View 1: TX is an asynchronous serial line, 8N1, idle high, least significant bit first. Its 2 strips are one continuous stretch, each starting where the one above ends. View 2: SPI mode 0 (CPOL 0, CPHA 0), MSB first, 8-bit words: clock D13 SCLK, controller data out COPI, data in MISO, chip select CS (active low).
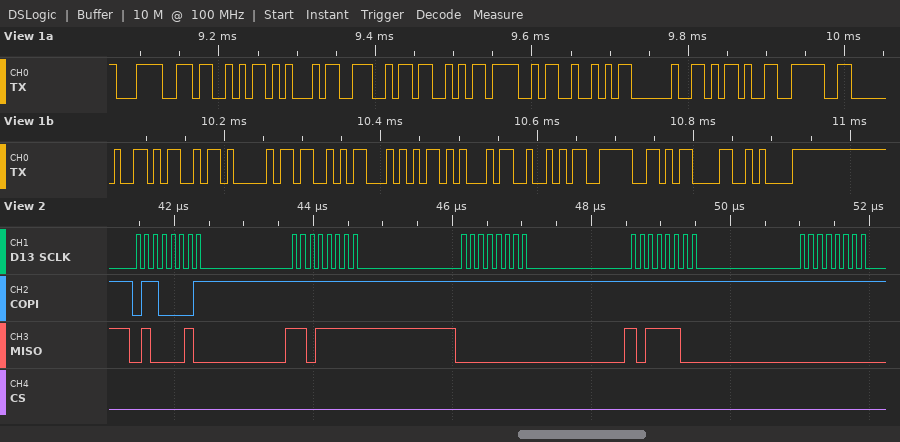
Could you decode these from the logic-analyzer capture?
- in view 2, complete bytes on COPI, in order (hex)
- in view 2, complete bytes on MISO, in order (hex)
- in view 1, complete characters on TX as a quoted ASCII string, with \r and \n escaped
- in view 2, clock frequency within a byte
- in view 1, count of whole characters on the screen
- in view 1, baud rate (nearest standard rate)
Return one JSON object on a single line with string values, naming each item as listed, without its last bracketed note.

{"in view 2, complete bytes on COPI, in order": "61 FF FF FF FF", "in view 2, complete bytes on MISO, in order": "42 DF 00 BC 00", "in view 1, complete characters on TX as a quoted ASCII string, with \\r and \\n escaped": "\"<SENSOR -> MASTER>\\r\\n\"", "in view 2, clock frequency within a byte": "8 MHz", "in view 1, count of whole characters on the screen": "20", "in view 1, baud rate": "115200 baud"}
